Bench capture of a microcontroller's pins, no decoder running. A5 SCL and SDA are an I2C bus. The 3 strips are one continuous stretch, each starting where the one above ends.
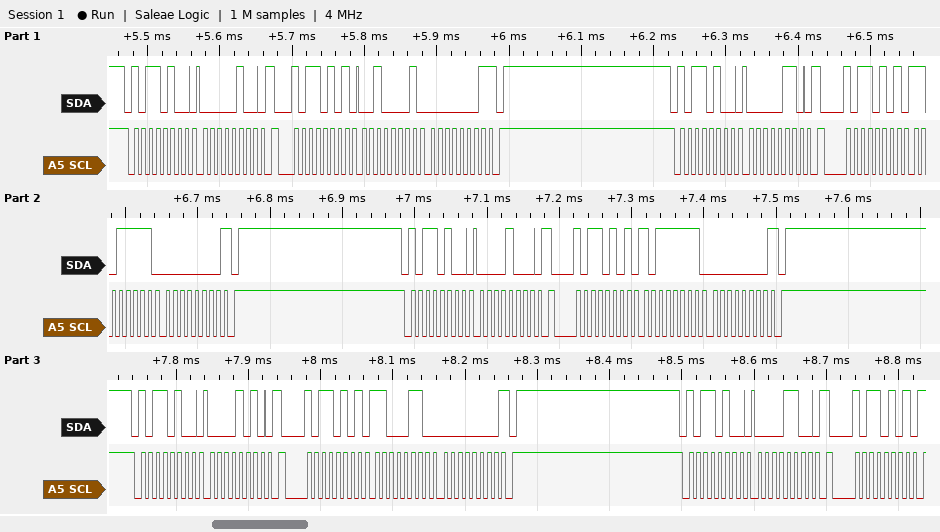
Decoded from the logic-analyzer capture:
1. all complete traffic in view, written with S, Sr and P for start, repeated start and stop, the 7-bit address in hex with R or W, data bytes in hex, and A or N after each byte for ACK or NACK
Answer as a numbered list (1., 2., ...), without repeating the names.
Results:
1. S 5AW A 04 A Sr 5AR A 21 A 01 N P S 5AW A 06 A Sr 5AR A DF A 00 N P S 5AW A 08 A Sr 5AR A BF A 00 N P S 5AW A 0A A Sr 5AR A C6 A 00 N P S 5AW A 0C A Sr 5AR A
